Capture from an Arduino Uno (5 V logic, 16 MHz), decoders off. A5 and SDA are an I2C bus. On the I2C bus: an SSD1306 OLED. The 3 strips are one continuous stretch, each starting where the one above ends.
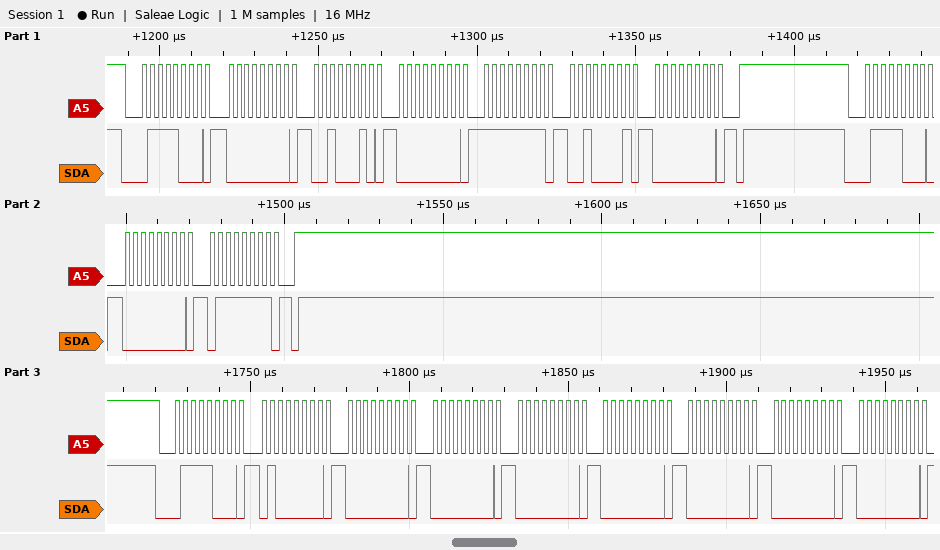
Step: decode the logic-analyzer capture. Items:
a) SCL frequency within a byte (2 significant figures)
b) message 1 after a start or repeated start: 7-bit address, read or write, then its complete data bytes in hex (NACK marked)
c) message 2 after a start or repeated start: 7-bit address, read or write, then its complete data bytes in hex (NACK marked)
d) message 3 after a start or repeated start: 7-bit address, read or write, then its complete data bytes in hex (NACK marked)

400 kHz
0x3C write: 00 22 00 FF 21 00
0x3C write: 00 7F
0x3C write: 40 00 00 00 00 00 00 00
